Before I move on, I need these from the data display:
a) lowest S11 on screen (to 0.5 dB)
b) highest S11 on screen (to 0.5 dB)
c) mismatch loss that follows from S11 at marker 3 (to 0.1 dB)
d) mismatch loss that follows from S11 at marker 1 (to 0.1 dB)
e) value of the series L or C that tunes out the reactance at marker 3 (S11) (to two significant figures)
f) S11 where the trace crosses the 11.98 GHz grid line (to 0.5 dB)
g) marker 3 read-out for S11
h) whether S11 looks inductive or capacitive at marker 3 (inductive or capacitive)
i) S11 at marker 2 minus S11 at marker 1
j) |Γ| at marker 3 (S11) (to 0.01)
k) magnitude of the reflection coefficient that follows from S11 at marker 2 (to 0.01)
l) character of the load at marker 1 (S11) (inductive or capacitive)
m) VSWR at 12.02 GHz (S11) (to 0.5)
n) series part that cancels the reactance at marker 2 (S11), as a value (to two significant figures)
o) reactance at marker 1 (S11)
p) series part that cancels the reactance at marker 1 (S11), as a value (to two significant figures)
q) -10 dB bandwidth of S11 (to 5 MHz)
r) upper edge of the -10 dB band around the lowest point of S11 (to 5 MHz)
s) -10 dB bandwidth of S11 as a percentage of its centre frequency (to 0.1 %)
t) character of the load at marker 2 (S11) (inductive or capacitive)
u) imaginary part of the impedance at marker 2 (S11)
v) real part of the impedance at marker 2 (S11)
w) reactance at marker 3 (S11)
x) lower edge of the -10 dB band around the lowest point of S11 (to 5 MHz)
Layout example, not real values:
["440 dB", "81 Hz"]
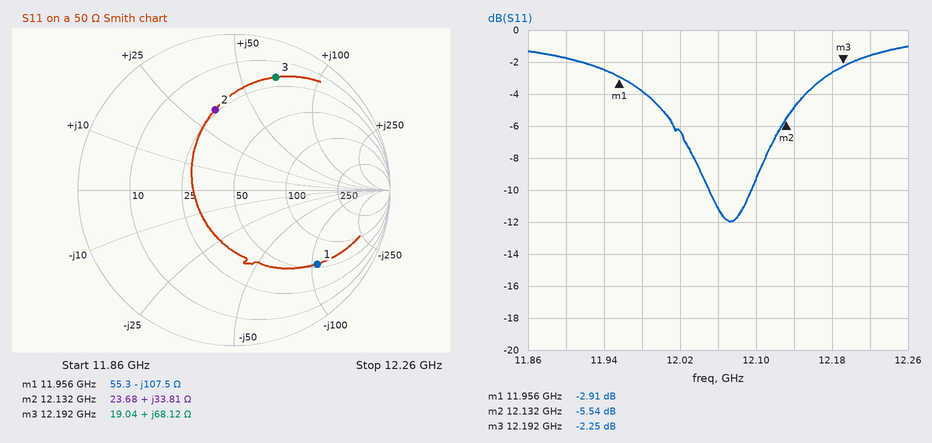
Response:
["-12.0 dB", "-1.0 dB", "3.9 dB", "3.1 dB", "190 fF", "-4.0 dB", "-2.25 dB", "inductive", "-2.63 dB", "0.77", "0.53", "capacitive", "3.0", "390 fF", "-107.5 Ω", "1.4 nH", "45 MHz", "12.095 GHz", "0.4 %", "inductive", "+33.81 Ω", "23.68 Ω", "+68.12 Ω", "12.050 GHz"]
